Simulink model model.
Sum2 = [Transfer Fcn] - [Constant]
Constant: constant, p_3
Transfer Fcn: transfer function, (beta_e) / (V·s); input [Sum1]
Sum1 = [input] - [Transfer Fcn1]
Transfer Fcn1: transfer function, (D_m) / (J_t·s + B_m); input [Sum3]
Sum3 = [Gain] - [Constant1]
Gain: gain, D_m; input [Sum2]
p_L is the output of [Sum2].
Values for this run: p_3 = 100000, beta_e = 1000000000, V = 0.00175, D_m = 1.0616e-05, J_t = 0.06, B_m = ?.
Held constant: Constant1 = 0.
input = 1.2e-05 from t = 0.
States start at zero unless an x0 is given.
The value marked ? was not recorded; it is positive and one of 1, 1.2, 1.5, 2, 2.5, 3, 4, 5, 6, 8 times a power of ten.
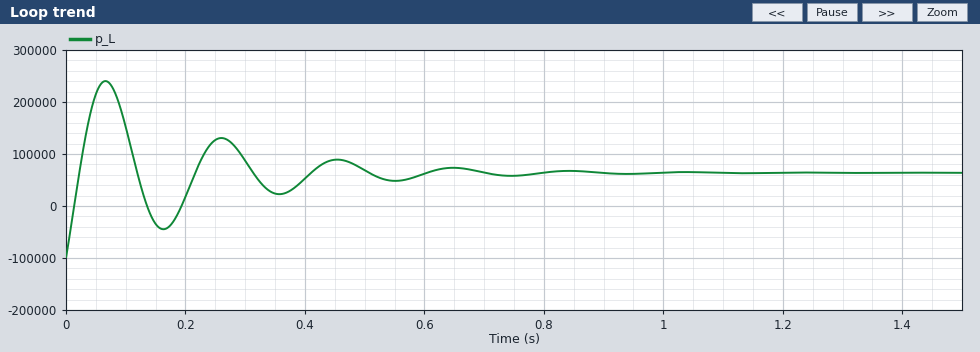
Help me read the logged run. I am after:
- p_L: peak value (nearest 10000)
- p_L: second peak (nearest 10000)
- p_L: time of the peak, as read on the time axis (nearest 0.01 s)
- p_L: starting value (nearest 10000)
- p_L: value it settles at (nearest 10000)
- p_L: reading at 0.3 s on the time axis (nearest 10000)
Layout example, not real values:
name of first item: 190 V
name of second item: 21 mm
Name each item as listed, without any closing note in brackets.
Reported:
p_L: peak value: 240000
p_L: second peak: 130000
p_L: time of the peak, as read on the time axis: 0.07 s
p_L: starting value: -100000
p_L: value it settles at: 60000
p_L: reading at 0.3 s on the time axis: 90000
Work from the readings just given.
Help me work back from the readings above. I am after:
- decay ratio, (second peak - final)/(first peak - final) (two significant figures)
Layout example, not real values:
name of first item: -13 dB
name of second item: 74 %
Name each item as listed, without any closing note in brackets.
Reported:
decay ratio, (second peak - final)/(first peak - final): 0.39
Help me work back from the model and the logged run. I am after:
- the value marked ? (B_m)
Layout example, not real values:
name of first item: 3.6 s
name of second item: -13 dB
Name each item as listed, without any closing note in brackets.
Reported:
the value marked ?: 0.6
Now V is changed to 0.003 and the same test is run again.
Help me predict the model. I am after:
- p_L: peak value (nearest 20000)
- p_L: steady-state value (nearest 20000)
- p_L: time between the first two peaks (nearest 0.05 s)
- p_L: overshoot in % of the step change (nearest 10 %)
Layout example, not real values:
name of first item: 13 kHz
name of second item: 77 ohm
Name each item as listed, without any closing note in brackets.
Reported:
p_L: peak value: 200000
p_L: steady-state value: 60000
p_L: time between the first two peaks: 0.25 s
p_L: overshoot in % of the step change: 80 %
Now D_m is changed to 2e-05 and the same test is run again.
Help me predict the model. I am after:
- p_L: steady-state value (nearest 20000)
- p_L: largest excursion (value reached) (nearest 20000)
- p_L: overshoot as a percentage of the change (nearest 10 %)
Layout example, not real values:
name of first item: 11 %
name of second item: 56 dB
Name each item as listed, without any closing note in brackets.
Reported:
p_L: steady-state value: 20000
p_L: largest excursion (value reached): 140000
p_L: overshoot as a percentage of the change: 110 %
